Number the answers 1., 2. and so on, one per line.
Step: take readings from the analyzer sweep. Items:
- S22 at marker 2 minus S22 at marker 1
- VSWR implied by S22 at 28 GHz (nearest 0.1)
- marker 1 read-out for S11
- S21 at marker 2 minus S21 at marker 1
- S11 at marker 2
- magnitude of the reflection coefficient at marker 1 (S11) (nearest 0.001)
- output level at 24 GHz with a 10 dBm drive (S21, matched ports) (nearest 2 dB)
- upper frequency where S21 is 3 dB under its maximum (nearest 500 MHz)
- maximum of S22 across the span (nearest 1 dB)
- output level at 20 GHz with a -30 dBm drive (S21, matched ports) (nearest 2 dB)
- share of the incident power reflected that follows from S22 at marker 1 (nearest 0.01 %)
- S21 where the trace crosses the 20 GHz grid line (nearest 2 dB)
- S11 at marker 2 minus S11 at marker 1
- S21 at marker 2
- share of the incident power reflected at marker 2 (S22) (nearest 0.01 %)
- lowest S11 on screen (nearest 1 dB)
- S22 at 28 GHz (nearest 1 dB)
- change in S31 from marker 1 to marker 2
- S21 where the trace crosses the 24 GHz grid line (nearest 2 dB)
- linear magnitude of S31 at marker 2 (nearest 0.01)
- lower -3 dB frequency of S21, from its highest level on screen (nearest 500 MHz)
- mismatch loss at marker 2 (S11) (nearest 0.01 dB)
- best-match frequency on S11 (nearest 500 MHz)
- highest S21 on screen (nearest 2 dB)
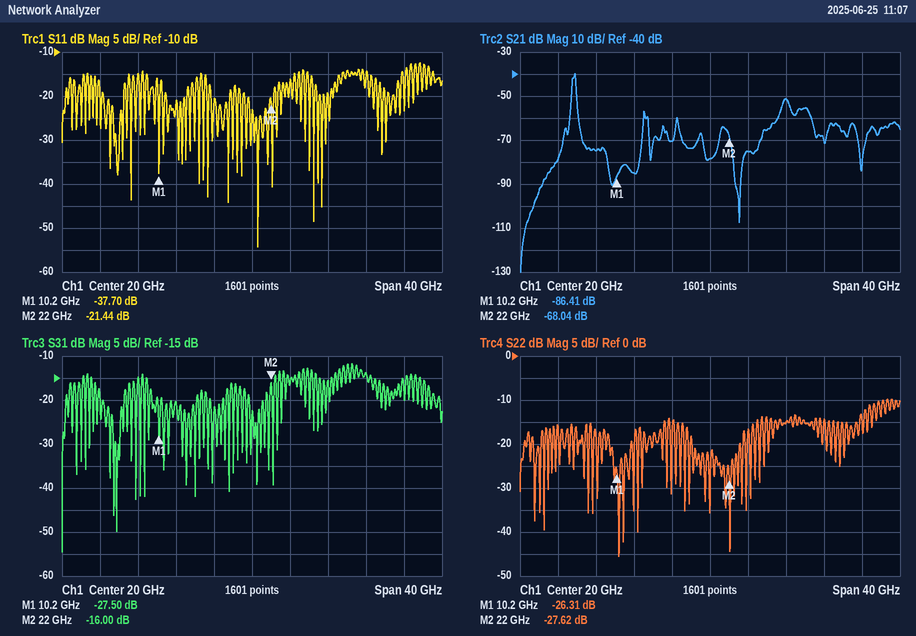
1. -1.31 dB
2. 1.4
3. -37.70 dB
4. 18.37 dB
5. -21.44 dB
6. 0.013
7. -66 dBm
8. 6.0 GHz
9. -10 dB
10. -108 dBm
11. 0.23 %
12. -78 dB
13. 16.26 dB
14. -68.04 dB
15. 0.17 %
16. -54 dB
17. -15 dB
18. 11.50 dB
19. -76 dB
20. 0.16
21. 5.5 GHz
22. 0.03 dB
23. 20.5 GHz
24. -40 dB
